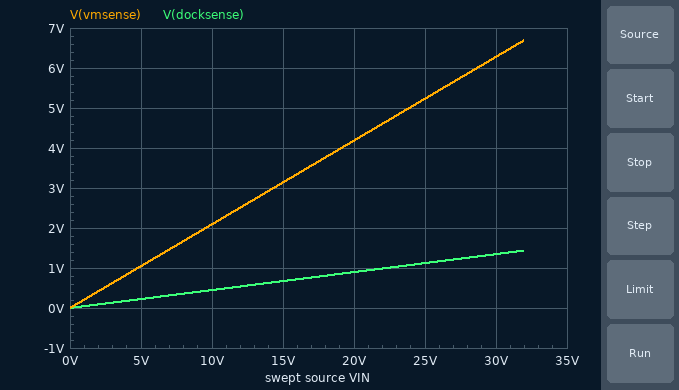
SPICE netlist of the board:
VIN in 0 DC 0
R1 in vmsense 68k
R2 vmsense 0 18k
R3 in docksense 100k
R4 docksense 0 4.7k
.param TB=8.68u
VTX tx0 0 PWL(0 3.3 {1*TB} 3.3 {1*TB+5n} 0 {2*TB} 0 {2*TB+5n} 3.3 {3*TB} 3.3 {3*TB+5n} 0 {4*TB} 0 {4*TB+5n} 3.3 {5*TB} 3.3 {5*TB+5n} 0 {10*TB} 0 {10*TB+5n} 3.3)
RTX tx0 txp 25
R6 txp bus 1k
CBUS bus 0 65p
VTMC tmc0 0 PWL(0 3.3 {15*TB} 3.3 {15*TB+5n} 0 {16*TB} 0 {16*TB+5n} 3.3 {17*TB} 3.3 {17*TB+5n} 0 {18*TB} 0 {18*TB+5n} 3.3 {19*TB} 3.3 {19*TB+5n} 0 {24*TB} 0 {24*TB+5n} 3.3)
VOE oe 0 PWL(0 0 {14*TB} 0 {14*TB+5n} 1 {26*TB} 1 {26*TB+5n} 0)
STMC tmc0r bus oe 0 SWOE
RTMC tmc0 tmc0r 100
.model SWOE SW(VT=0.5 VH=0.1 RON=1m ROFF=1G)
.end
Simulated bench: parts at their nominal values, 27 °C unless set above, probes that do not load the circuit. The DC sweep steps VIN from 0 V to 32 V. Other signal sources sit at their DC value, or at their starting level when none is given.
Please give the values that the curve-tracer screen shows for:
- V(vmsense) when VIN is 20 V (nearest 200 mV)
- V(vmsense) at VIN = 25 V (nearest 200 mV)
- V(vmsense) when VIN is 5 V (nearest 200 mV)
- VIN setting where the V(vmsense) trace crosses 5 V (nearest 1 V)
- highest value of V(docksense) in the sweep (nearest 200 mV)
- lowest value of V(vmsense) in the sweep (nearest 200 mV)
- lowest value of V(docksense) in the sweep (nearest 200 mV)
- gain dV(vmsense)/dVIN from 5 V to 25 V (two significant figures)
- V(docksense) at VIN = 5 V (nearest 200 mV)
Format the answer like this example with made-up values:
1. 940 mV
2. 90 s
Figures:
1. 4.2 V
2. 5.2 V
3. 1.0 V
4. 24 V
5. 1.4 V
6. 0 V
7. 0 V
8. 0.21 V/V
9. 200 mV
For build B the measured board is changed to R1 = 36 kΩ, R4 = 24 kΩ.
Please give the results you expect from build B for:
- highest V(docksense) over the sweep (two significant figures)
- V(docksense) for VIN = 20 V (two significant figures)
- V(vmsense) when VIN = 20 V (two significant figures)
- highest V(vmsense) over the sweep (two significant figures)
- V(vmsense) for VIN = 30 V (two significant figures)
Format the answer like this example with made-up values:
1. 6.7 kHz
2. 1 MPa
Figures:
1. 6.2 V
2. 3.9 V
3. 6.7 V
4. 11 V
5. 10 V
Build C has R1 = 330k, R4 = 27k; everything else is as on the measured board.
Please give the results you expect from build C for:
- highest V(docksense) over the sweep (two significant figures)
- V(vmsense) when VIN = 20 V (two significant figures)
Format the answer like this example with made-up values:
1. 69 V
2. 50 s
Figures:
1. 6.8 V
2. 1.0 V
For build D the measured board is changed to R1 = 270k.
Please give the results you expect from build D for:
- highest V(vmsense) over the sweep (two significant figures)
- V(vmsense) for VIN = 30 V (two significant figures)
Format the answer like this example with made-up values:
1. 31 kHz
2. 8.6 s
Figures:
1. 2.0 V
2. 1.9 V
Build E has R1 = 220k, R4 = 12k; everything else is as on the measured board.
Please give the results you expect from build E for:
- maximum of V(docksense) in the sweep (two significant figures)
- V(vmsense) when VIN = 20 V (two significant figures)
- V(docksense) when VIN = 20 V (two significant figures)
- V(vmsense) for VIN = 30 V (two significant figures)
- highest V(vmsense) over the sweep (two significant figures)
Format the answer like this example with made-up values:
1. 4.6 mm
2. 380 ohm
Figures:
1. 3.4 V
2. 1.5 V
3. 2.1 V
4. 2.3 V
5. 2.4 V
